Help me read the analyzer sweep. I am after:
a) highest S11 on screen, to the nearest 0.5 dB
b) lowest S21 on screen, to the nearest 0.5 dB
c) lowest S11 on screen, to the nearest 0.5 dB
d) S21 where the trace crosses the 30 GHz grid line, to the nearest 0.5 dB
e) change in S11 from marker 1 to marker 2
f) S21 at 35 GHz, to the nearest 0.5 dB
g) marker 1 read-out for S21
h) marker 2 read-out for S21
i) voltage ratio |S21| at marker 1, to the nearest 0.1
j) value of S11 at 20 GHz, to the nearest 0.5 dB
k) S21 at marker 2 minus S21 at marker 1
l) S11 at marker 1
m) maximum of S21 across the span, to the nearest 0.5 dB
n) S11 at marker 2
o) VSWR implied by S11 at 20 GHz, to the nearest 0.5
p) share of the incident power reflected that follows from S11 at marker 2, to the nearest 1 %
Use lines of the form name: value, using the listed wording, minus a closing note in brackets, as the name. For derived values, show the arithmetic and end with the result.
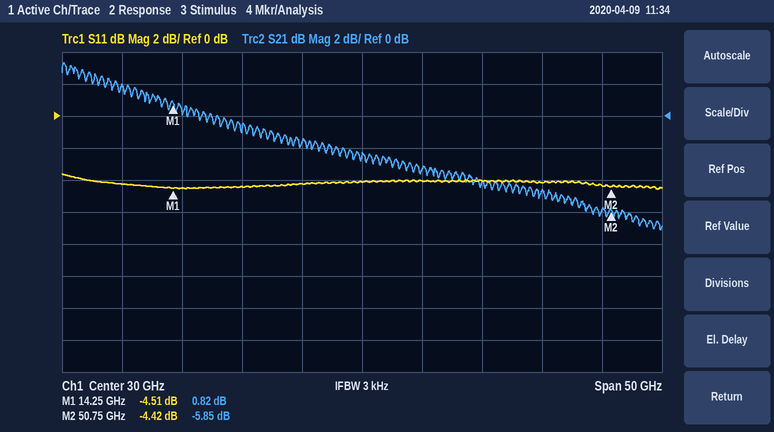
highest S11 on screen, to the nearest 0.5 dB: -3.5 dB
lowest S21 on screen, to the nearest 0.5 dB: -7.0 dB
lowest S11 on screen, to the nearest 0.5 dB: -4.5 dB
S21 where the trace crosses the 30 GHz grid line, to the nearest 0.5 dB: -2.5 dB
change in S11 from marker 1 to marker 2: -4.42 − (-4.51) = 0.09 dB
S21 at 35 GHz, to the nearest 0.5 dB: -3.5 dB
marker 1 read-out for S21: 0.82 dB
marker 2 read-out for S21: -5.85 dB
voltage ratio |S21| at marker 1, to the nearest 0.1: 10^(0.82/20) ≈ 1.1
value of S11 at 20 GHz, to the nearest 0.5 dB: -4.5 dB
S21 at marker 2 minus S21 at marker 1: -5.85 − (0.82) = -6.67 dB
S11 at marker 1: -4.51 dB
maximum of S21 across the span, to the nearest 0.5 dB: 3.5 dB
S11 at marker 2: -4.42 dB
VSWR implied by S11 at 20 GHz, to the nearest 0.5: |Γ| = 10^(-4.5/20) = 0.5957; VSWR = (1 + 0.5957)/(1 − 0.5957) ≈ 4.0
share of the incident power reflected that follows from S11 at marker 2, to the nearest 1 %: 10^(-4.42/10) ≈ 36 %
